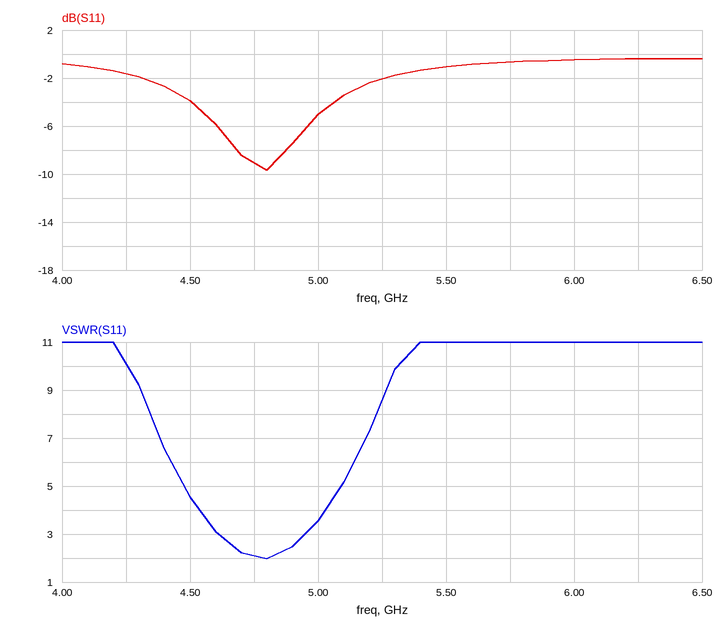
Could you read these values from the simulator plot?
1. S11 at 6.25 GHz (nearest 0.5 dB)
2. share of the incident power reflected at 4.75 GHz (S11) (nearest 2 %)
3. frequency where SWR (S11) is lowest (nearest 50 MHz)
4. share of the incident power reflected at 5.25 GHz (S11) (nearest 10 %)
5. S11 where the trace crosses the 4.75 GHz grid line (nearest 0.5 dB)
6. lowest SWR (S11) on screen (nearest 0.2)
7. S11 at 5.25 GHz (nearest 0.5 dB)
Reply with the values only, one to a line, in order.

-0.5 dB
12 %
4.80 GHz
60 %
-9.0 dB
2.0
-2.0 dB
